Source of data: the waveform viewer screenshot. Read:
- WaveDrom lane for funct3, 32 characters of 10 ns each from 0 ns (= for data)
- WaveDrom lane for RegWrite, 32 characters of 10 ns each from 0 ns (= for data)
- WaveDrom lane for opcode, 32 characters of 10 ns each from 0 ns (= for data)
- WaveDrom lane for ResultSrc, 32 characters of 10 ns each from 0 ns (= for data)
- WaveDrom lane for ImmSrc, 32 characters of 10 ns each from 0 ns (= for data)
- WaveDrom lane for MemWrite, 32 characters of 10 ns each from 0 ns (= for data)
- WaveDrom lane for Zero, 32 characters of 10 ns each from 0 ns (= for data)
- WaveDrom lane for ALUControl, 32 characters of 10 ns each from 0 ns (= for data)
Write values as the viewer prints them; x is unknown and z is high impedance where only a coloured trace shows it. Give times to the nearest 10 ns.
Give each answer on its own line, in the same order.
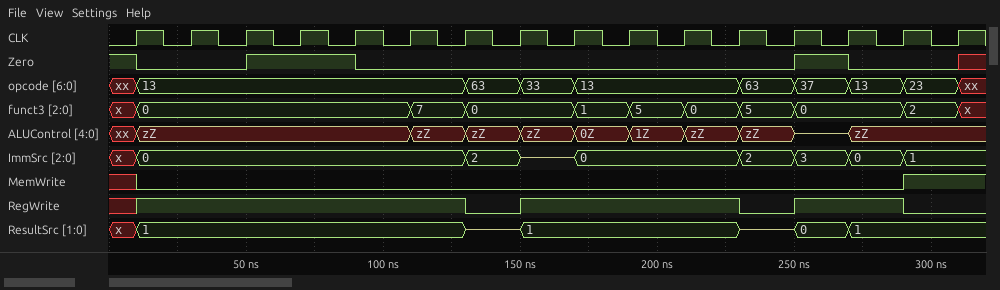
{name: 'funct3', wave: 'x=.........=.=...=.=.=.=.=...=.x', data: '0 7 0 1 5 0 5 0 2'}
{name: 'RegWrite', wave: 'x1...........0.1.......0.1...0..'}
{name: 'opcode', wave: 'x=...........=.=.=.....=.=.=.=.x', data: '13 63 33 13 63 37 13 23'}
{name: 'ResultSrc', wave: 'x=...........z.=.......z.=.=....', data: '1 1 0 1'}
{name: 'ImmSrc', wave: 'x=...........=.z.=.....=.=.=.=..', data: '0 2 0 2 3 0 1'}
{name: 'MemWrite', wave: 'x0...........................1..'}
{name: 'Zero', wave: '10...1...0...............1.0...x'}
{name: 'ALUControl', wave: 'x=.........=.=.=.=.=.=.=.z.=....', data: 'zZ zZ zZ zZ 0Z 1Z zZ zZ zZ'}
